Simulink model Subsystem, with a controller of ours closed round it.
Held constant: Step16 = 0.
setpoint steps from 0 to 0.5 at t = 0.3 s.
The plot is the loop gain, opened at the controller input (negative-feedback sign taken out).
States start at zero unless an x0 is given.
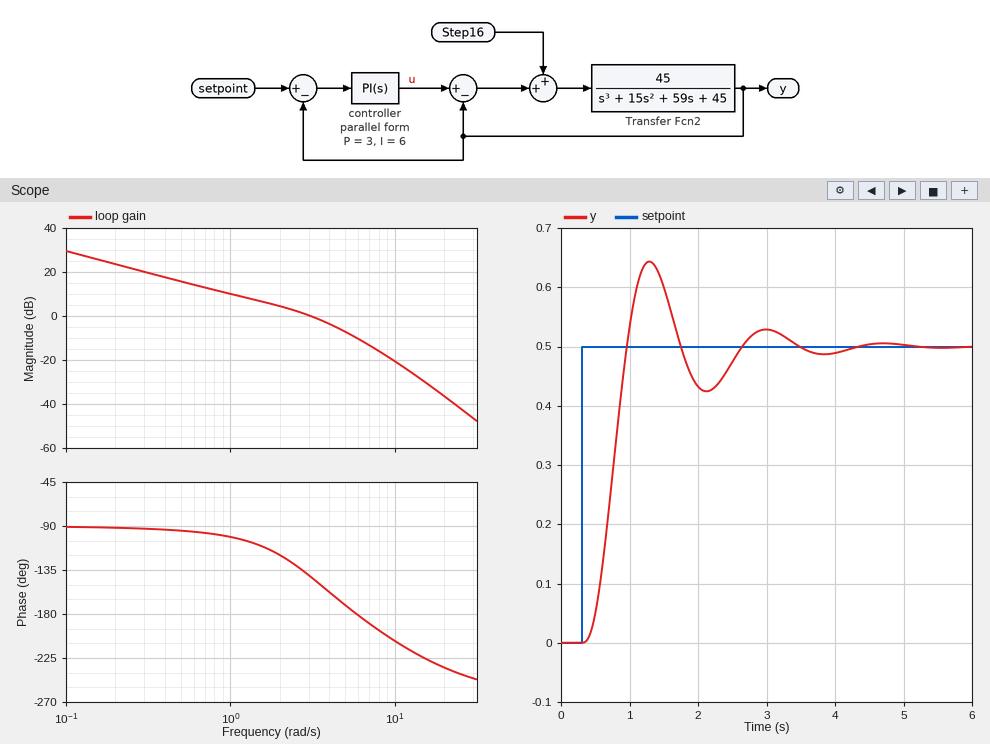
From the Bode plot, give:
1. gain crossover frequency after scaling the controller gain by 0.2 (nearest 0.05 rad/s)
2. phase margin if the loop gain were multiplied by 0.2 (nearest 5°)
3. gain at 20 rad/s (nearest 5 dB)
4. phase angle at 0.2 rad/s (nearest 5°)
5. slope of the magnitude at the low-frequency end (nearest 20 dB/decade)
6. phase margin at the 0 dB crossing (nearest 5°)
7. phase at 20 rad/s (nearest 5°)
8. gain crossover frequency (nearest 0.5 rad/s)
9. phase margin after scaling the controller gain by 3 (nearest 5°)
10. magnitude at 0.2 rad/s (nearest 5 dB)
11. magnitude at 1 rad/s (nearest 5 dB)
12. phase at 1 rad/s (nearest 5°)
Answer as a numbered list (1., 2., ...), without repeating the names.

1. 0.60 rad/s
2. 85°
3. -35 dB
4. -90°
5. -20 dB/decade
6. 40°
7. -235°
8. 3.0 rad/s
9. 0°
10. 25 dB
11. 10 dB
12. -100°
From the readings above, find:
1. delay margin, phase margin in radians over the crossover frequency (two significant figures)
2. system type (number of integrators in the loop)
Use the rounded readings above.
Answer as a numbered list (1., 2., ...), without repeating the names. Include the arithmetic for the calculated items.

1. 40 × π / 180 / 3 = 0.23 s
2. 1
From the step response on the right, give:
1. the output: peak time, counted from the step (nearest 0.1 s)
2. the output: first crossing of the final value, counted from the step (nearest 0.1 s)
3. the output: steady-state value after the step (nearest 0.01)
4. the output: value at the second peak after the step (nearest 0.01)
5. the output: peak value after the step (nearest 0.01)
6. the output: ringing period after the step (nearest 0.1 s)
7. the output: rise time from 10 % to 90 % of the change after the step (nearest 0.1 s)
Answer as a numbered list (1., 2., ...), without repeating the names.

1. 1.0 s
2. 0.7 s
3. 0.50
4. 0.53
5. 0.64
6. 1.7 s
7. 0.4 s
